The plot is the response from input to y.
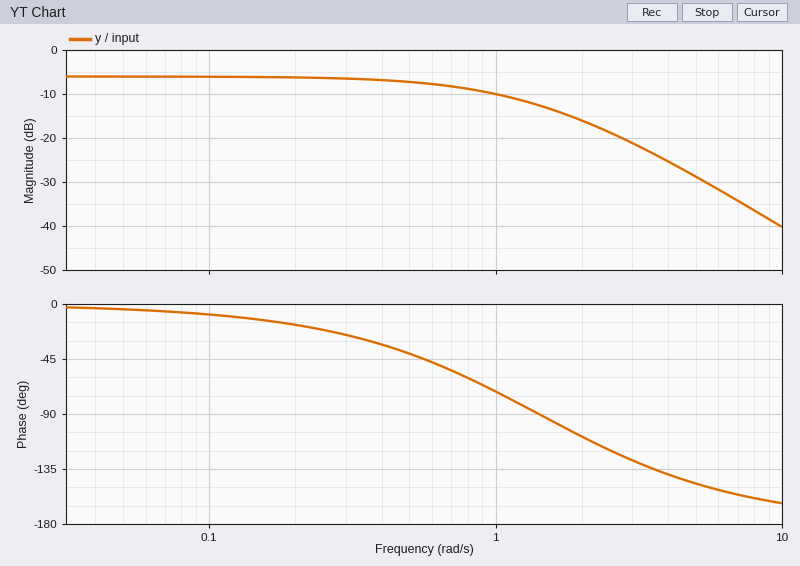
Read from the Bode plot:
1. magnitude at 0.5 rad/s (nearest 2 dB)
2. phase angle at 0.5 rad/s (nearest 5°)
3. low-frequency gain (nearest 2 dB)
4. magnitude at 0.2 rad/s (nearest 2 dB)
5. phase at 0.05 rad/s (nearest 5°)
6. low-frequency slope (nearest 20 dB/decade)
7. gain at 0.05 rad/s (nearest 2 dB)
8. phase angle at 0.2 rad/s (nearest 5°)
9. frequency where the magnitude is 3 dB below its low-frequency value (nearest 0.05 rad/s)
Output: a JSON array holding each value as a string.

["-8 dB", "-40°", "-6 dB", "-6 dB", "-5°", "0 dB/decade", "-6 dB", "-15°", "0.85 rad/s"]
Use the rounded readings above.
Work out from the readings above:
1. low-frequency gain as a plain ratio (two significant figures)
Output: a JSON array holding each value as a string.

["0.50"]
